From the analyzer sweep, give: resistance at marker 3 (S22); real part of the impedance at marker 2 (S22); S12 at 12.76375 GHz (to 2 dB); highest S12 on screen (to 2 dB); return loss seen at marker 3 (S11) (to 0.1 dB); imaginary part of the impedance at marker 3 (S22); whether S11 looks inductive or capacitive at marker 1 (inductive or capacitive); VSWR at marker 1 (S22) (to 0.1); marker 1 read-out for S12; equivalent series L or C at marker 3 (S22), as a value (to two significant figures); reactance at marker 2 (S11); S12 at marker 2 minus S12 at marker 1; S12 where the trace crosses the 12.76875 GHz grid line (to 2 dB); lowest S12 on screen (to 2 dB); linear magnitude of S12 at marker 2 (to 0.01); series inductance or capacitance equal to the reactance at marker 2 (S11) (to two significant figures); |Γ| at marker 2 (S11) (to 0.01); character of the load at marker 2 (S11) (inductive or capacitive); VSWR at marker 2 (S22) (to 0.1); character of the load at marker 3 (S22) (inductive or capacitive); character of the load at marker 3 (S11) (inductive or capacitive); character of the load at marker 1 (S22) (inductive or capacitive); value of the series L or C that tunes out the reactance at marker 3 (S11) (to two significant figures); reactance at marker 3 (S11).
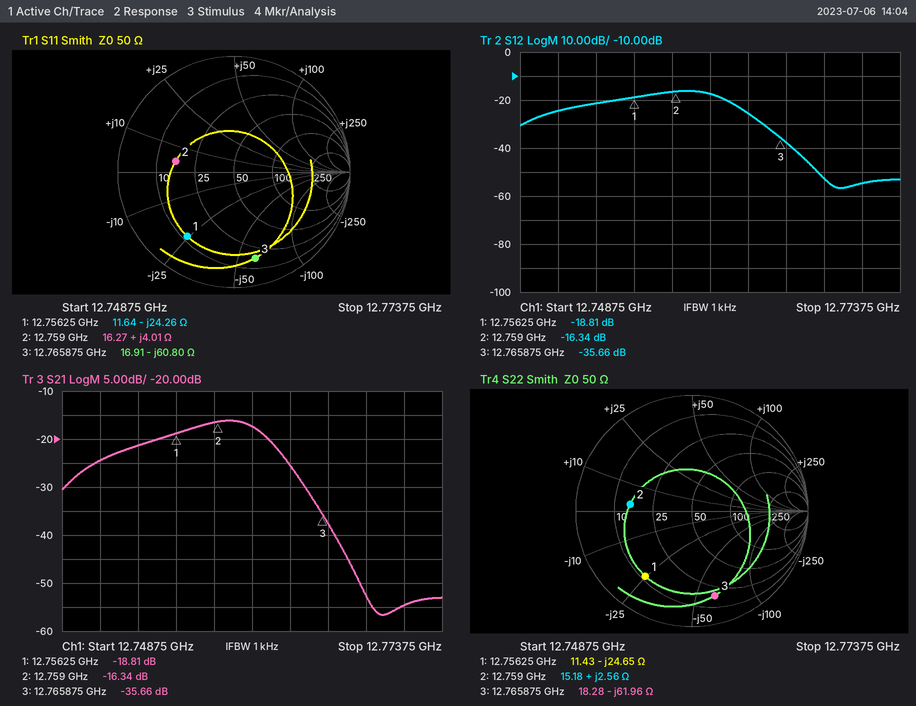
18.28 Ω
15.18 Ω
-26 dB
-16 dB
2.3 dB
-61.96 Ω
capacitive
5.5
-18.81 dB
200 fF
+4.01 Ω
2.47 dB
-52 dB
-56 dB
0.15
50 pH
0.51
inductive
3.3
capacitive
capacitive
capacitive
760 pH
-60.80 Ω
